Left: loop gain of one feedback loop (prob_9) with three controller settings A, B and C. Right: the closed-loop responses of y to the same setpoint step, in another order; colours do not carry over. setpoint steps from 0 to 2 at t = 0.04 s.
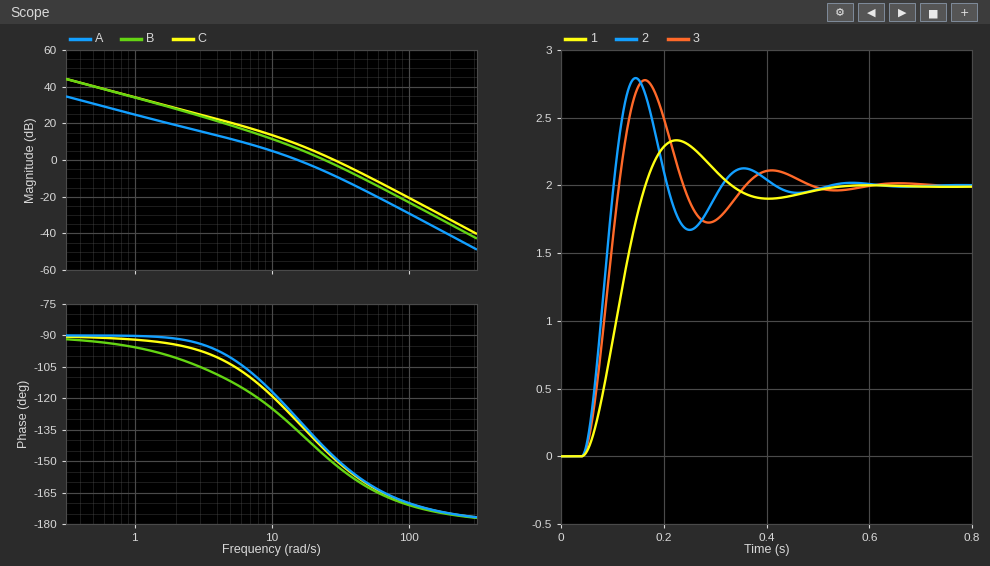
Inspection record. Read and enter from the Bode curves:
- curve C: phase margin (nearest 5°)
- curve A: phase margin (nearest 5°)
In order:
30°
50°
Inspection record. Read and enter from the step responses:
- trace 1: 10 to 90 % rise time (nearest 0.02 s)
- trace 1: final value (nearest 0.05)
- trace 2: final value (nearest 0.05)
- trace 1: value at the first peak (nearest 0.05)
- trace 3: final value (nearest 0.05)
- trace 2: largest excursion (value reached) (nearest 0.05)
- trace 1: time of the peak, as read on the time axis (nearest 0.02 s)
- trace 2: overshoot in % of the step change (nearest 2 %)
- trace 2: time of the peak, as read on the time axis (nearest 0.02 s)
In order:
0.08 s
2.00
2.00
2.35
2.00
2.80
0.22 s
40 %
0.14 s
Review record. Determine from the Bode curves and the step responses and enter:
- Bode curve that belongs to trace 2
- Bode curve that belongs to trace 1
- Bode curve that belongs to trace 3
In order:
C
A
B
